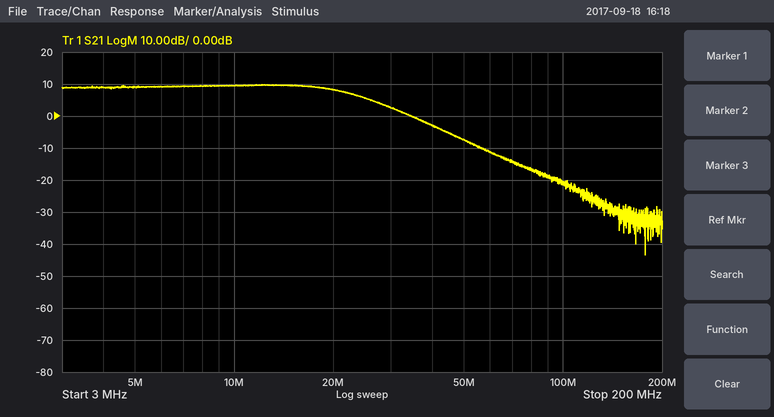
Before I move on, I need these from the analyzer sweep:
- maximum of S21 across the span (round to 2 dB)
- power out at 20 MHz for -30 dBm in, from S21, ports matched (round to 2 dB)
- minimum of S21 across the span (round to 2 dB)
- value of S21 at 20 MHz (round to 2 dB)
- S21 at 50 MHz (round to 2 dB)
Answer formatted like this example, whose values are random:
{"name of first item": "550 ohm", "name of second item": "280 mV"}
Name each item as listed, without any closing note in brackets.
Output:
{"maximum of S21 across the span": "10 dB", "power out at 20 MHz for -30 dBm in, from S21, ports matched": "-22 dBm", "minimum of S21 across the span": "-44 dB", "value of S21 at 20 MHz": "8 dB", "S21 at 50 MHz": "-8 dB"}
